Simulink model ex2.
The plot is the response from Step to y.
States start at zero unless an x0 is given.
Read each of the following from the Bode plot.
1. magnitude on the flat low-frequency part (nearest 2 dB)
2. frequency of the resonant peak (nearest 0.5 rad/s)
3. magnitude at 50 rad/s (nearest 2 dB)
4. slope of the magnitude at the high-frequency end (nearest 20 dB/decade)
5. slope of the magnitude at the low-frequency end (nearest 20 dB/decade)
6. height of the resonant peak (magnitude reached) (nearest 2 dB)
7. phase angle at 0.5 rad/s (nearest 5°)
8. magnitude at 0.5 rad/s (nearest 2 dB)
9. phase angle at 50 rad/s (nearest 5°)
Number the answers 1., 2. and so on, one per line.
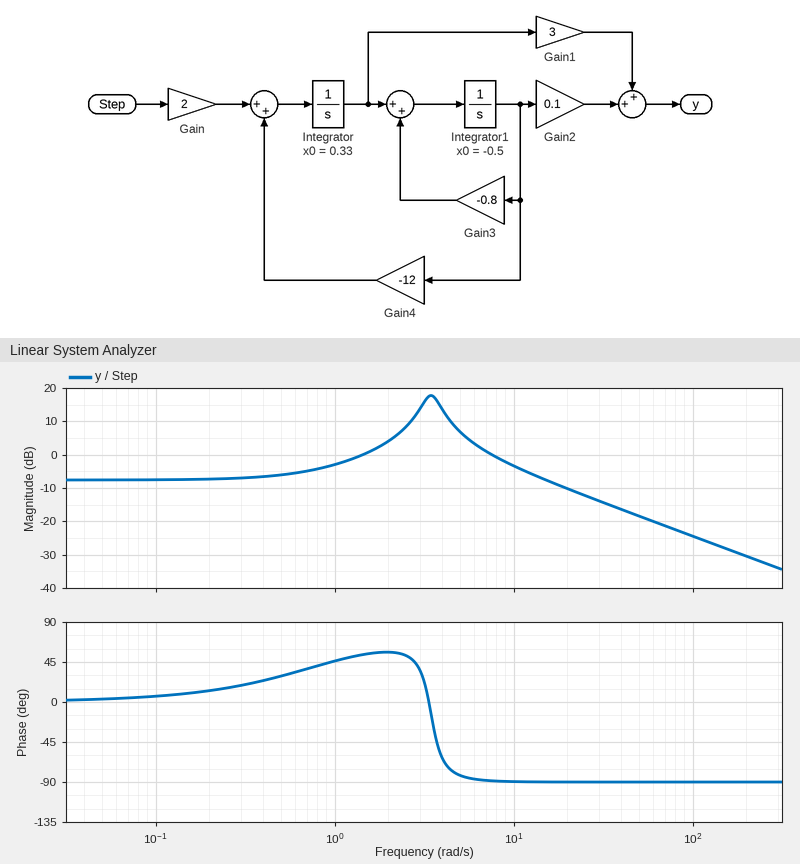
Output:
1. -8 dB
2. 3.5 rad/s
3. -18 dB
4. -20 dB/decade
5. 0 dB/decade
6. 18 dB
7. 30°
8. -6 dB
9. -90°
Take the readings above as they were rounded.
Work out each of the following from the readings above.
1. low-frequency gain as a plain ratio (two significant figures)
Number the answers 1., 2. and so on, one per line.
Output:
1. 0.40
